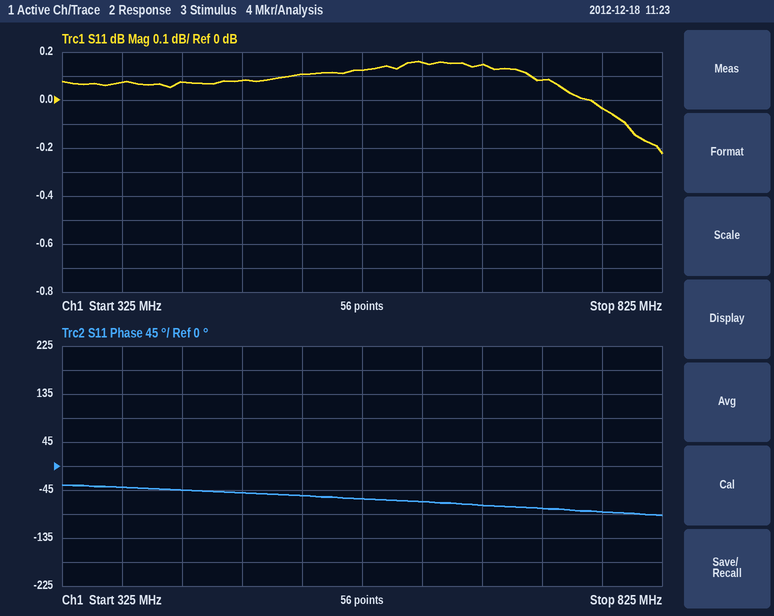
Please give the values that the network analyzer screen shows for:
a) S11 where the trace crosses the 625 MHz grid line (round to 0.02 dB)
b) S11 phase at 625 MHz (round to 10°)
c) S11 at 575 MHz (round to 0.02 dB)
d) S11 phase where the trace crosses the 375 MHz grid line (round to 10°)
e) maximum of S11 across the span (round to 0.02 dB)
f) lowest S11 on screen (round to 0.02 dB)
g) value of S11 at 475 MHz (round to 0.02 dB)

0.16 dB
-70°
0.12 dB
-40°
0.16 dB
-0.22 dB
0.08 dB
